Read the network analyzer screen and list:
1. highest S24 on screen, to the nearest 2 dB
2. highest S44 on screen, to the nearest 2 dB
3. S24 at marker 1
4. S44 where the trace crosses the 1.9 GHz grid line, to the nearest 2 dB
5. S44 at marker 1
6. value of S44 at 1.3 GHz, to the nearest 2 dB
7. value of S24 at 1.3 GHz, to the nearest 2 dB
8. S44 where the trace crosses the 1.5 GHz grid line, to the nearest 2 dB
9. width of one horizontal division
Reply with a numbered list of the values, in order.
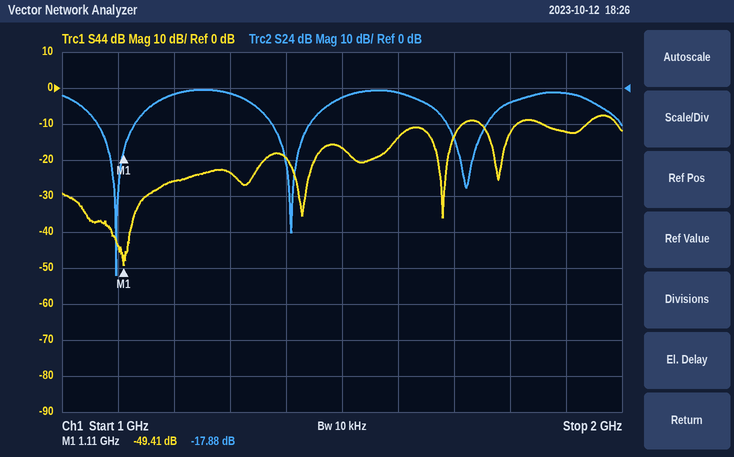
1. 0 dB
2. -8 dB
3. -17.88 dB
4. -12 dB
5. -49.41 dB
6. -24 dB
7. -2 dB
8. -16 dB
9. 100 MHz
